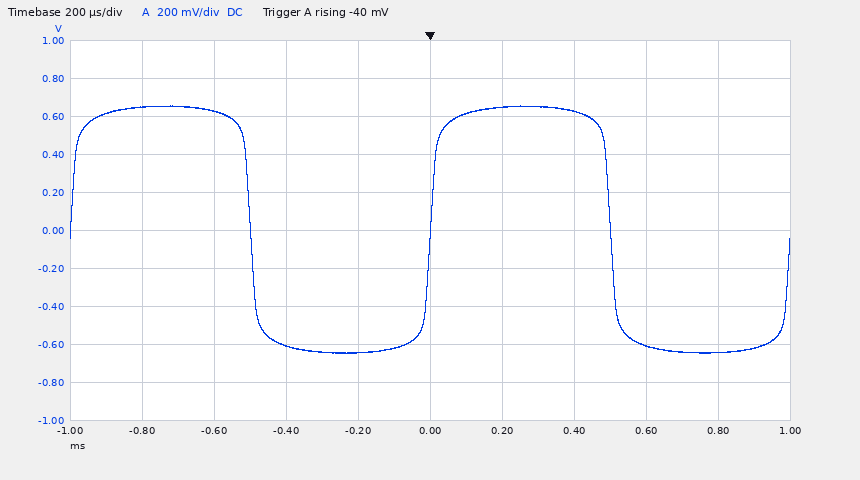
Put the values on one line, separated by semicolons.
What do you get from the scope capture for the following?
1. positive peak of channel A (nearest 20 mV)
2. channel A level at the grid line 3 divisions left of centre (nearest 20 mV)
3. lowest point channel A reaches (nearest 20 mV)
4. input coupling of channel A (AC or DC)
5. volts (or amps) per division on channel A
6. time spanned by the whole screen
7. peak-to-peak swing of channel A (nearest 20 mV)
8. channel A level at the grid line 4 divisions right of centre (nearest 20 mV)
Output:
660 mV; 620 mV; -640 mV; DC; 200 mV; 2 ms; 1.30 V; -640 mV
